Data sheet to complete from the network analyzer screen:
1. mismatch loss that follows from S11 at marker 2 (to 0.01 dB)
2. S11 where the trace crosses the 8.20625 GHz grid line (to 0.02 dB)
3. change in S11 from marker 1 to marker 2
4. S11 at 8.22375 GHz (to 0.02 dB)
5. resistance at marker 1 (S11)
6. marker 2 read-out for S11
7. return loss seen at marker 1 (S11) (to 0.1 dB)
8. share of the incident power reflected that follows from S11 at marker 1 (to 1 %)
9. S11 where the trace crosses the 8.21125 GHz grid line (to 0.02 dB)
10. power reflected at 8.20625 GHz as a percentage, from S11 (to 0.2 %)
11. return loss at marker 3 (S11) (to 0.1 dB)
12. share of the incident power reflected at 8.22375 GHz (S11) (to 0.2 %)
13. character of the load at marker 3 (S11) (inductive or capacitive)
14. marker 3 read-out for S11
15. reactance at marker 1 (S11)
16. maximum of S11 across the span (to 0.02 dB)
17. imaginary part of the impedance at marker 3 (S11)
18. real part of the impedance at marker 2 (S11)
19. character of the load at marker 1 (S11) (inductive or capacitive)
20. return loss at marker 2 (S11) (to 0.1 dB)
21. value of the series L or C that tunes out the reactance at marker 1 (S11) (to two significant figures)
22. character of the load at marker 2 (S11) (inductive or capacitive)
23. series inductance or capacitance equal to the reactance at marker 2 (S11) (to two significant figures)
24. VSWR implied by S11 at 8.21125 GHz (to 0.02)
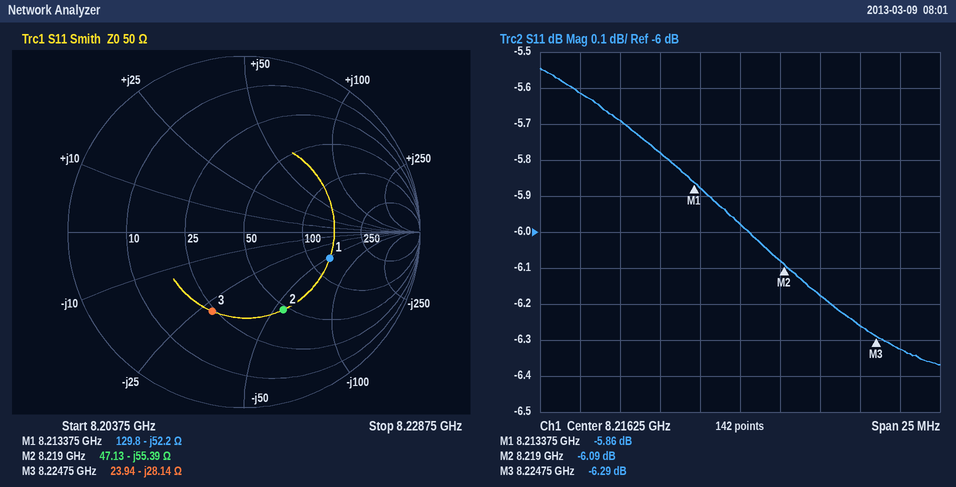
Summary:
1.23 dB
-5.62 dB
-0.23 dB
-6.26 dB
129.8 Ω
-6.09 dB
5.9 dB
26 %
-5.78 dB
27.4 %
6.3 dB
23.6 %
capacitive
-6.29 dB
-52.2 Ω
-5.54 dB
-28.14 Ω
47.13 Ω
capacitive
6.1 dB
1.0 nH
capacitive
350 fF
3.12
